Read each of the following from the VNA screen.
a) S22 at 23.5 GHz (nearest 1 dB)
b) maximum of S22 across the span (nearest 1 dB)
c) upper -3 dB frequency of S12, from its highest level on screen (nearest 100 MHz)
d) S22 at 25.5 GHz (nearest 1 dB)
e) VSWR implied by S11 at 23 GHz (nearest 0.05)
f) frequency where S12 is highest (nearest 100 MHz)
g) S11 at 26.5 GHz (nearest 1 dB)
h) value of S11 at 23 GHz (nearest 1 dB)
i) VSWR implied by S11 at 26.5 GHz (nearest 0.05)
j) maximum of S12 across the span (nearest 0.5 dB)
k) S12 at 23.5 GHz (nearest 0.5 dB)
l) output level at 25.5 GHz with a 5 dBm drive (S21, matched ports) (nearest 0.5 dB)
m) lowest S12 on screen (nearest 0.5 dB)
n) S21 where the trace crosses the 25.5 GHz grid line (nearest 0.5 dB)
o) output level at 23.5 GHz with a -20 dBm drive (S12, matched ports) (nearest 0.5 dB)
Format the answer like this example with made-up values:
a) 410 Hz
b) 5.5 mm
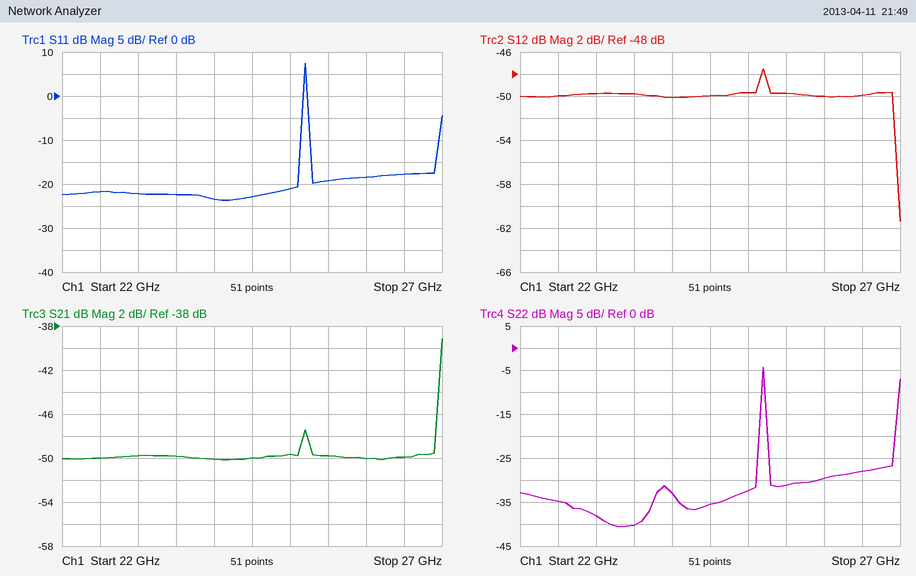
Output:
a) -40 dB
b) -4 dB
c) 26.9 GHz
d) -31 dB
e) 1.15
f) 25.2 GHz
g) -18 dB
h) -22 dB
i) 1.30
j) -47.5 dB
k) -50.0 dB
l) -45.0 dBm
m) -61.5 dB
n) -50.0 dB
o) -70.0 dBm
